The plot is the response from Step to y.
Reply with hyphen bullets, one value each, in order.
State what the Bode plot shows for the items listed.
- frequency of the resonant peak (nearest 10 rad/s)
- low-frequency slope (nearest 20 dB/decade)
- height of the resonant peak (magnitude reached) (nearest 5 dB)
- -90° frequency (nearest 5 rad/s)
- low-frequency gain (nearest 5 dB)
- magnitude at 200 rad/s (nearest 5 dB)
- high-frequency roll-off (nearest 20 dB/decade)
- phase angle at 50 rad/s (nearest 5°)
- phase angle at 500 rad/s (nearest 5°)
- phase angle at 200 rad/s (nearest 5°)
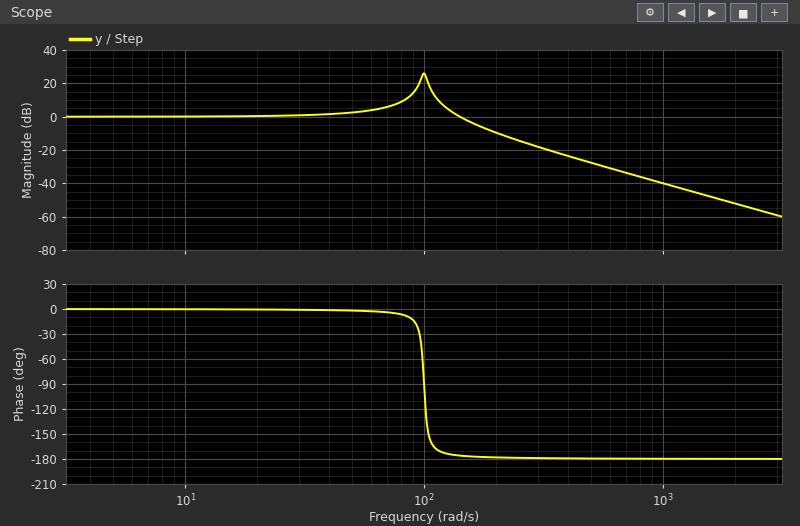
- 100 rad/s
- 0 dB/decade
- 25 dB
- 100 rad/s
- 0 dB
- -10 dB
- -40 dB/decade
- 0°
- -180°
- -180°
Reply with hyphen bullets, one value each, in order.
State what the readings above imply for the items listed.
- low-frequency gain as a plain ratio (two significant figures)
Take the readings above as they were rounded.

- 1.0
